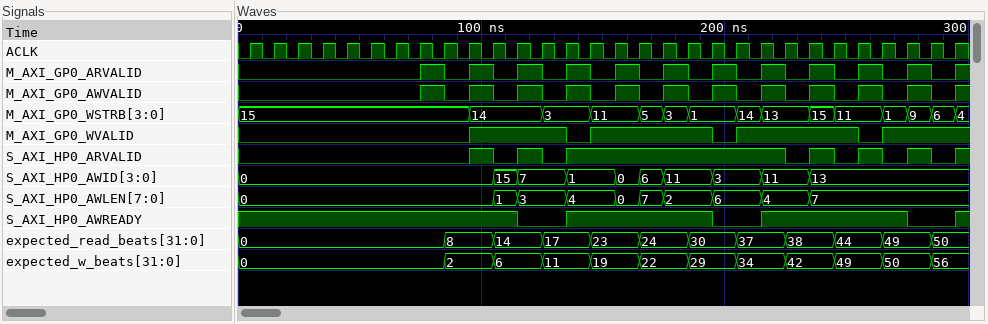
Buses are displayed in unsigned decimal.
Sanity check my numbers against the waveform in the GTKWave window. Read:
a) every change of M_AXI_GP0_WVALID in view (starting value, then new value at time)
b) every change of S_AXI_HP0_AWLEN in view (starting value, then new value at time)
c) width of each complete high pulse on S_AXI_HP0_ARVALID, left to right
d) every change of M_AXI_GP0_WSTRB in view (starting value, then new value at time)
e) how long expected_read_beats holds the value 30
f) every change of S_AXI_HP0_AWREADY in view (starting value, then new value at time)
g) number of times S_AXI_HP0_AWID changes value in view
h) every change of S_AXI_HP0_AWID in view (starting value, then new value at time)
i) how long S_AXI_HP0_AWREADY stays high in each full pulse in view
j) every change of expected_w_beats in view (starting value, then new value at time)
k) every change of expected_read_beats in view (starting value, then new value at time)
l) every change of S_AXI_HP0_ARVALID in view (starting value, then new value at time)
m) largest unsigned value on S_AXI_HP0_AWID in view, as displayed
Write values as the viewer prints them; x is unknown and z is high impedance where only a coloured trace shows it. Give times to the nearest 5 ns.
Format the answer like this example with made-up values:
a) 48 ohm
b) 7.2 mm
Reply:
a) 0, 1 at 95 ns, 0 at 135 ns, 1 at 145 ns, 0 at 195 ns, 1 at 205 ns, 0 at 255 ns, 1 at 265 ns
b) 0, 1 at 105 ns, 3 at 115 ns, 4 at 135 ns, 0 at 155 ns, 7 at 165 ns, 2 at 175 ns, 6 at 195 ns, 4 at 215 ns, 7 at 235 ns
c) 10 ns, 10 ns, 90 ns, 10 ns, 10 ns, 10 ns
d) 15, 14 at 95 ns, 3 at 125 ns, 11 at 145 ns, 5 at 165 ns, 3 at 175 ns, 1 at 185 ns, 14 at 205 ns, 13 at 215 ns, 15 at 235 ns, 11 at 245 ns, 1 at 265 ns, 9 at 275 ns, 6 at 285 ns, 4 at 295 ns
e) 20 ns
f) 1, 0 at 115 ns, 1 at 135 ns, 0 at 195 ns, 1 at 215 ns, 0 at 275 ns, 1 at 295 ns
g) 9
h) 0, 15 at 105 ns, 7 at 115 ns, 1 at 135 ns, 0 at 155 ns, 6 at 165 ns, 11 at 175 ns, 3 at 195 ns, 11 at 215 ns, 13 at 235 ns
i) 60 ns, 60 ns
j) 0, 2 at 85 ns, 6 at 105 ns, 11 at 125 ns, 19 at 145 ns, 22 at 165 ns, 29 at 185 ns, 34 at 205 ns, 42 at 225 ns, 49 at 245 ns, 50 at 265 ns, 56 at 285 ns
k) 0, 8 at 85 ns, 14 at 105 ns, 17 at 125 ns, 23 at 145 ns, 24 at 165 ns, 30 at 185 ns, 37 at 205 ns, 38 at 225 ns, 44 at 245 ns, 49 at 265 ns, 50 at 285 ns
l) 0, 1 at 95 ns, 0 at 105 ns, 1 at 115 ns, 0 at 125 ns, 1 at 135 ns, 0 at 225 ns, 1 at 235 ns, 0 at 245 ns, 1 at 255 ns, 0 at 265 ns, 1 at 275 ns, 0 at 285 ns, 1 at 295 ns
m) 15
